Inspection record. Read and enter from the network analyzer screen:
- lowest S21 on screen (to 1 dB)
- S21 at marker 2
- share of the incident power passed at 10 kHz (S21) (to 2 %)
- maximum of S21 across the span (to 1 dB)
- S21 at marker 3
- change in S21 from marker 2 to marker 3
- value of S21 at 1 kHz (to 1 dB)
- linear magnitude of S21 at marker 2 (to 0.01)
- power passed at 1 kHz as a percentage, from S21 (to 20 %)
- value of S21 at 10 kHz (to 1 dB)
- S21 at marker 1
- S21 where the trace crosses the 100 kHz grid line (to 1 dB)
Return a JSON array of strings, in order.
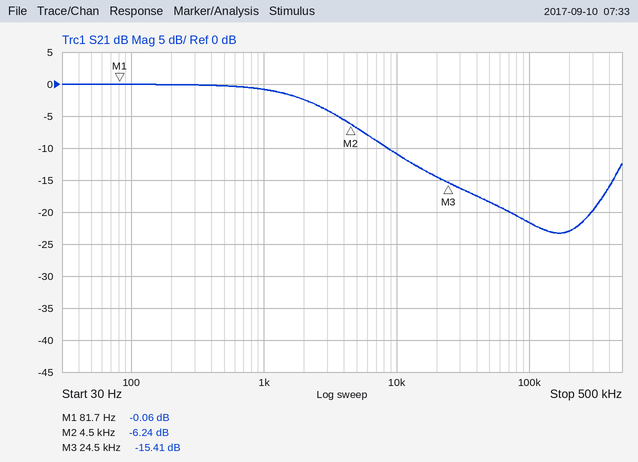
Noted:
["-23 dB", "-6.24 dB", "8 %", "0 dB", "-15.41 dB", "-9.17 dB", "-1 dB", "0.49", "80 %", "-11 dB", "-0.06 dB", "-22 dB"]
